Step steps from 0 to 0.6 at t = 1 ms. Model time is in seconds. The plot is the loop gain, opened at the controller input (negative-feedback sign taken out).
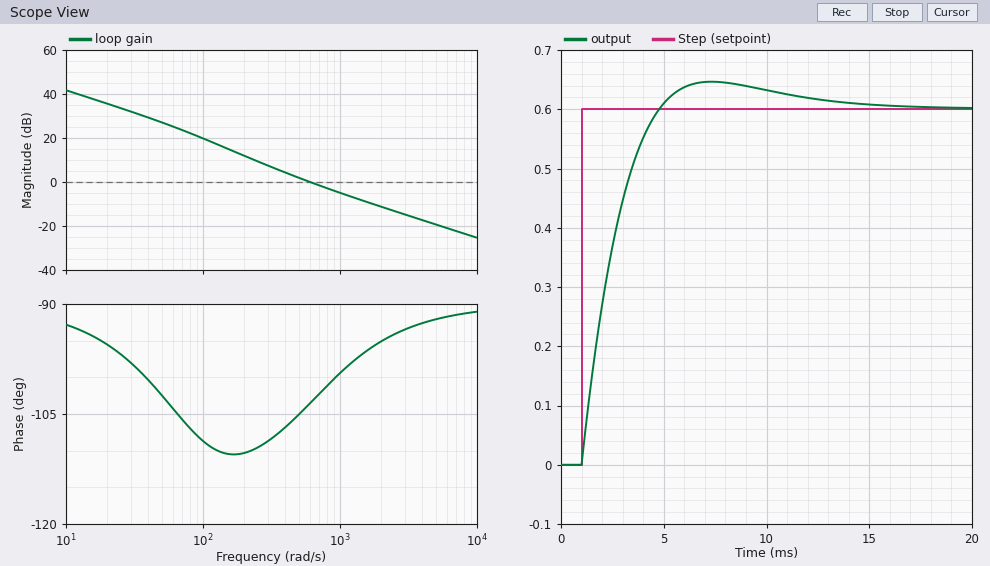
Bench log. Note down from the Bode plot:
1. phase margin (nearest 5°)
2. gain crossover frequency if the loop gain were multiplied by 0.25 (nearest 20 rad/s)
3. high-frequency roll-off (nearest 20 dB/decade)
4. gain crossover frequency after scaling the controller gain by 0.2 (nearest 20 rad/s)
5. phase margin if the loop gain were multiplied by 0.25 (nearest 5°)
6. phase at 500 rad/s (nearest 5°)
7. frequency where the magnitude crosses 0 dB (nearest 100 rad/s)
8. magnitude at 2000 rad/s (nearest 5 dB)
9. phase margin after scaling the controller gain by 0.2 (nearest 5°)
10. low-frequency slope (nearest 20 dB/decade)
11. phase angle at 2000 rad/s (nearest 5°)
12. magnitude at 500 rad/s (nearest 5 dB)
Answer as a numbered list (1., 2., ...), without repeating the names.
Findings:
1. 75°
2. 200 rad/s
3. -20 dB/decade
4. 160 rad/s
5. 70°
6. -105°
7. 600 rad/s
8. -10 dB
9. 70°
10. -20 dB/decade
11. -95°
12. 0 dB
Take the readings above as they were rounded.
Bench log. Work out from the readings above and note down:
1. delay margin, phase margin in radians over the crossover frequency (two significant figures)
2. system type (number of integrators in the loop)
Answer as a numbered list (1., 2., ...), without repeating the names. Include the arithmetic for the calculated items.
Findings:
1. 75 × π / 180 / 600 = 0.0022 s
2. 1
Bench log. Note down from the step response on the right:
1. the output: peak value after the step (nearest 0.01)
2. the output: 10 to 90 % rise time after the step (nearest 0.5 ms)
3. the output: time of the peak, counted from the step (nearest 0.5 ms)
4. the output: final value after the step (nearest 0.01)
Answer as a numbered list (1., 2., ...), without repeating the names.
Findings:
1. 0.65
2. 2.5 ms
3. 6.5 ms
4. 0.60
